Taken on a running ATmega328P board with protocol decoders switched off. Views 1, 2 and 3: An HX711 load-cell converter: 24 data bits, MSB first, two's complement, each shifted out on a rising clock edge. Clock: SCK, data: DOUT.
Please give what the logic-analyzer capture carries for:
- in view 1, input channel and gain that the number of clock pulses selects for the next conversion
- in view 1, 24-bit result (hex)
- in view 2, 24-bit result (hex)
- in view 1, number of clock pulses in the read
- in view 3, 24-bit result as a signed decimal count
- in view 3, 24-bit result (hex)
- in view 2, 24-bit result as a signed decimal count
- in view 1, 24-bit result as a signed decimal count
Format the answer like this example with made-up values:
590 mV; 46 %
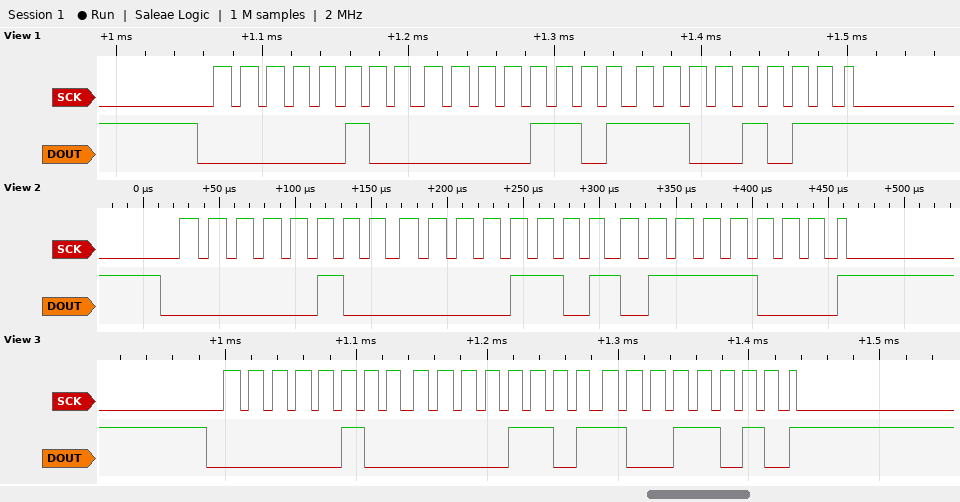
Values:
channel A, gain 128; 0x040DCB; 0x040D78; 25; 265626; 0x040D9A; 265592; 265675
